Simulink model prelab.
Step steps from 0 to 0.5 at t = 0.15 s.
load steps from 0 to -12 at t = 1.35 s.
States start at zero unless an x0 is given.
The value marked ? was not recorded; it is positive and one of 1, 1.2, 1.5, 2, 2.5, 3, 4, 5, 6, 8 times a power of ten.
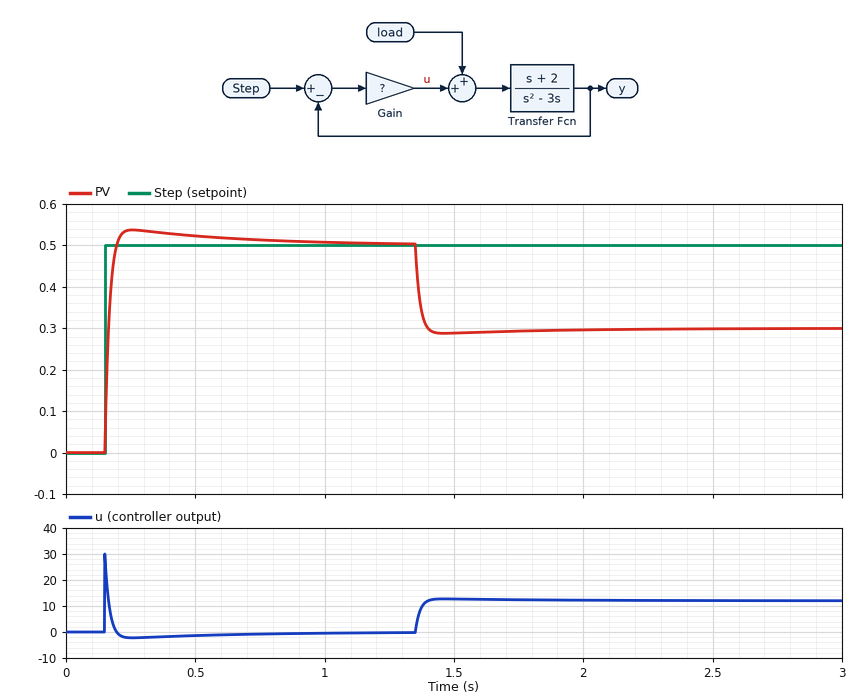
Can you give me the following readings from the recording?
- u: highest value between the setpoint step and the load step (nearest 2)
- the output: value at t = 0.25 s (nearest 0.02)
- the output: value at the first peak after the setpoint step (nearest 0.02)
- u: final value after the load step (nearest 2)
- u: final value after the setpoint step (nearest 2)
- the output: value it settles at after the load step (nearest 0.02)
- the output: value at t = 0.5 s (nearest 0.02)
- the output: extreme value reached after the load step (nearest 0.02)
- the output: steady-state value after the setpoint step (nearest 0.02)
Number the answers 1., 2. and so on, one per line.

1. 30
2. 0.54
3. 0.54
4. 12
5. 0
6. 0.30
7. 0.52
8. 0.28
9. 0.50
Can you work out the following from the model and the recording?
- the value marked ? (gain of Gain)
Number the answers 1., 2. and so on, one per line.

1. 60
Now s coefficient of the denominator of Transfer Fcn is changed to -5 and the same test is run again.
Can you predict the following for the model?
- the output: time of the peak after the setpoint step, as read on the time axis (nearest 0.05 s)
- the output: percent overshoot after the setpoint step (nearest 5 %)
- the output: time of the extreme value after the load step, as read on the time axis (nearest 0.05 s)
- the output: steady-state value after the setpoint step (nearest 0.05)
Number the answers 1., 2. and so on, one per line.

1. 0.25 s
2. 10 %
3. 1.45 s
4. 0.50
